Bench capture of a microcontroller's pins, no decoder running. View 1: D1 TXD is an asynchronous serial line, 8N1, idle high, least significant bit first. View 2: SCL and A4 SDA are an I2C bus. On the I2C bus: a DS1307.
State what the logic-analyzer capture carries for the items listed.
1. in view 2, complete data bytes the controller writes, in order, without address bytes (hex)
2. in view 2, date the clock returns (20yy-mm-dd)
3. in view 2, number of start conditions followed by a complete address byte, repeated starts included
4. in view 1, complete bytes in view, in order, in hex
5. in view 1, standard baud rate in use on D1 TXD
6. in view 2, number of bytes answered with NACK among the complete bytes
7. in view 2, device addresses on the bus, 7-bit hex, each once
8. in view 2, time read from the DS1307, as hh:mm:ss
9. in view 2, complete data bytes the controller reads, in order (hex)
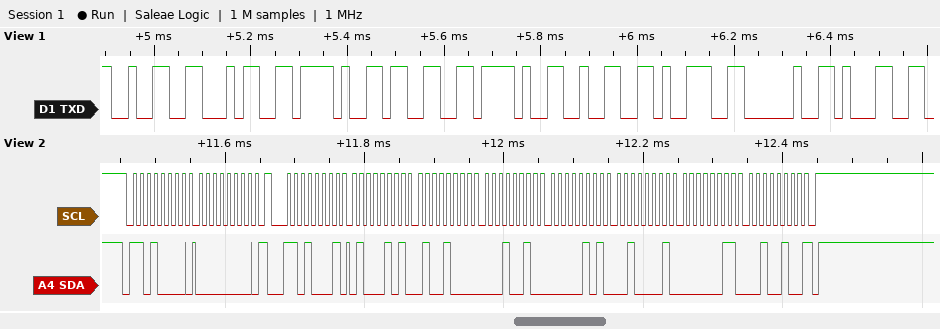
00
2024-03-21
2
32 34 2F 33 2F 32 39 20 31
57600 baud
1
0x68
12:48:45
45 48 12 05 21 03 24
